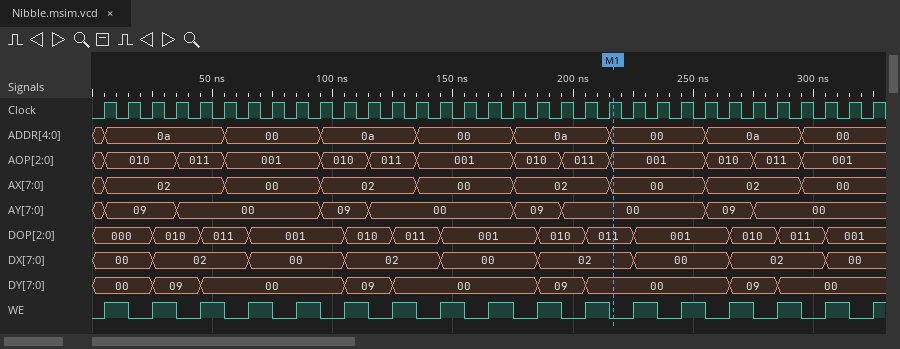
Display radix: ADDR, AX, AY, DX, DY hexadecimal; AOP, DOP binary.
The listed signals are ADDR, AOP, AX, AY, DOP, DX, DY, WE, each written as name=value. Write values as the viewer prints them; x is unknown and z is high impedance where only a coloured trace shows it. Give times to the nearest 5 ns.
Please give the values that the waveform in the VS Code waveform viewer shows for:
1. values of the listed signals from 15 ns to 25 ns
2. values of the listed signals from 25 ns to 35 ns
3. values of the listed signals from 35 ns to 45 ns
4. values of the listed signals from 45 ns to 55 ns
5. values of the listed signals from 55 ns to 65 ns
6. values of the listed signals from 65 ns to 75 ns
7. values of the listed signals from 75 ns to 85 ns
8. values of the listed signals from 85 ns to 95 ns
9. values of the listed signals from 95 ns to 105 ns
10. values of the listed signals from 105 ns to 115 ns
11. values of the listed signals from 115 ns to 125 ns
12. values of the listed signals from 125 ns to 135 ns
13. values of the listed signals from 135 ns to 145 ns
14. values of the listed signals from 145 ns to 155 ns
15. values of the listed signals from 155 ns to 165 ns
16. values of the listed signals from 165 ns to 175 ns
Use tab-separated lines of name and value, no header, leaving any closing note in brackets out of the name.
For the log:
values of the listed signals from 15 ns to 25 ns	ADDR=0a, AOP=010, AX=02, AY=09, DOP=000, DX=00, DY=00, WE=0
values of the listed signals from 25 ns to 35 ns	ADDR=0a, AOP=010, AX=02, AY=09, DOP=010, DX=02, DY=09, WE=1
values of the listed signals from 35 ns to 45 ns	ADDR=0a, AOP=011, AX=02, AY=00, DOP=010, DX=02, DY=09, WE=0
values of the listed signals from 45 ns to 55 ns	ADDR=0a, AOP=011, AX=02, AY=00, DOP=011, DX=02, DY=00, WE=1
values of the listed signals from 55 ns to 65 ns	ADDR=00, AOP=001, AX=00, AY=00, DOP=011, DX=02, DY=00, WE=0
values of the listed signals from 65 ns to 75 ns	ADDR=00, AOP=001, AX=00, AY=00, DOP=001, DX=00, DY=00, WE=1
values of the listed signals from 75 ns to 85 ns	ADDR=00, AOP=001, AX=00, AY=00, DOP=001, DX=00, DY=00, WE=0
values of the listed signals from 85 ns to 95 ns	ADDR=00, AOP=001, AX=00, AY=00, DOP=001, DX=00, DY=00, WE=1
values of the listed signals from 95 ns to 105 ns	ADDR=0a, AOP=010, AX=02, AY=09, DOP=001, DX=00, DY=00, WE=0
values of the listed signals from 105 ns to 115 ns	ADDR=0a, AOP=010, AX=02, AY=09, DOP=010, DX=02, DY=09, WE=1
values of the listed signals from 115 ns to 125 ns	ADDR=0a, AOP=011, AX=02, AY=00, DOP=010, DX=02, DY=09, WE=0
values of the listed signals from 125 ns to 135 ns	ADDR=0a, AOP=011, AX=02, AY=00, DOP=011, DX=02, DY=00, WE=1
values of the listed signals from 135 ns to 145 ns	ADDR=00, AOP=001, AX=00, AY=00, DOP=011, DX=02, DY=00, WE=0
values of the listed signals from 145 ns to 155 ns	ADDR=00, AOP=001, AX=00, AY=00, DOP=001, DX=00, DY=00, WE=1
values of the listed signals from 155 ns to 165 ns	ADDR=00, AOP=001, AX=00, AY=00, DOP=001, DX=00, DY=00, WE=0
values of the listed signals from 165 ns to 175 ns	ADDR=00, AOP=001, AX=00, AY=00, DOP=001, DX=00, DY=00, WE=1
